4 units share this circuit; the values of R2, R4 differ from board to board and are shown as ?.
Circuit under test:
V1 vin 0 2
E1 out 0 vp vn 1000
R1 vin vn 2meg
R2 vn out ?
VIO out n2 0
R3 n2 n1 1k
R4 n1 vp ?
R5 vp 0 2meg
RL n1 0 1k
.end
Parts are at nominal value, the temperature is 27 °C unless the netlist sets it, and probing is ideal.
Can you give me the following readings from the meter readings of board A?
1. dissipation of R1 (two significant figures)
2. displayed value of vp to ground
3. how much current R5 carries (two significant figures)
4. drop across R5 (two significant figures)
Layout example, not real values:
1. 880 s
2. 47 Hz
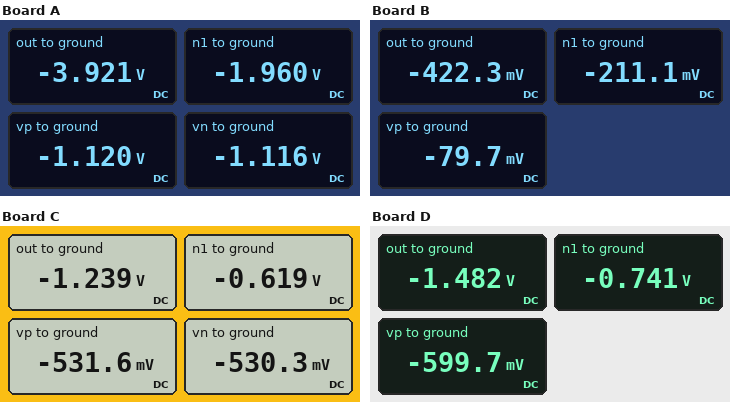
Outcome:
1. 4.9 µW
2. -1.120 V
3. 560 nA
4. 1.1 V
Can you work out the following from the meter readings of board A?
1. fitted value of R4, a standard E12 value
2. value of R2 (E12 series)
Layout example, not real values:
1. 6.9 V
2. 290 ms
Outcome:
1. 1.5 MΩ
2. 1.8 MΩ
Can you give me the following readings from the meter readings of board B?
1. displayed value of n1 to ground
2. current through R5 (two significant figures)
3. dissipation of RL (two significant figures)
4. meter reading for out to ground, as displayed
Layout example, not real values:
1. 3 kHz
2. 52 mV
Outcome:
1. -211.1 mV
2. 40 nA
3. 45 µW
4. -422.3 mV
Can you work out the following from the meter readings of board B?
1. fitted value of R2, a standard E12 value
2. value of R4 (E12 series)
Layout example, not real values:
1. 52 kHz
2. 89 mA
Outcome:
1. 330 kΩ
2. 3.3 MΩ
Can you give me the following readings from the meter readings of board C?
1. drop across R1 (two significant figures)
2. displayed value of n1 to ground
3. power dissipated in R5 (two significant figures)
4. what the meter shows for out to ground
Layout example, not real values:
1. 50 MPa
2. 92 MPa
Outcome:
1. 2.5 V
2. -0.619 V
3. 140 nW
4. -1.239 V
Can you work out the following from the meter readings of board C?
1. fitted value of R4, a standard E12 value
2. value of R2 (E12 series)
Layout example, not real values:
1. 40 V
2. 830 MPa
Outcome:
1. 330 kΩ
2. 560 kΩ
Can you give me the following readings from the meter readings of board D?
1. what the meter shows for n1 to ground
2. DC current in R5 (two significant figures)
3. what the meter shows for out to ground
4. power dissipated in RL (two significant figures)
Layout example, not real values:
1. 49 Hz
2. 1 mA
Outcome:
1. -0.741 V
2. 300 nA
3. -1.482 V
4. 550 µW
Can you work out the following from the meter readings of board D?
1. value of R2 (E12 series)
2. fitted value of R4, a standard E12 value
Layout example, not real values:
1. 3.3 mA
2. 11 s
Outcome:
1. 680 kΩ
2. 470 kΩ
